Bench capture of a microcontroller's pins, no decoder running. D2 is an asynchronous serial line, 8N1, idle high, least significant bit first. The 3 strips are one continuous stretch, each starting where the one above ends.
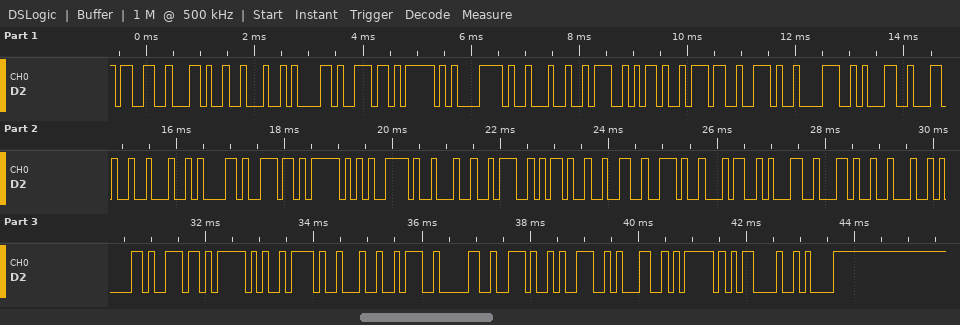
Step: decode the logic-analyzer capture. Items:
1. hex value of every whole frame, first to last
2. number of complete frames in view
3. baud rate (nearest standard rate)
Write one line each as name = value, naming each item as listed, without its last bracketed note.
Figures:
hex value of every whole frame, first to last = 33 2C 22 61 6E 5F 78 22 3A 2D 37 2E 38 31 2C 22 61 6E 5F 79 22 3A 2D 32 2E 34 31 2C 22 61 6E 5F 7A 22 3A 30 2E 39 31 7D 0D 0A
number of complete frames in view = 42
baud rate = 9600 baud
